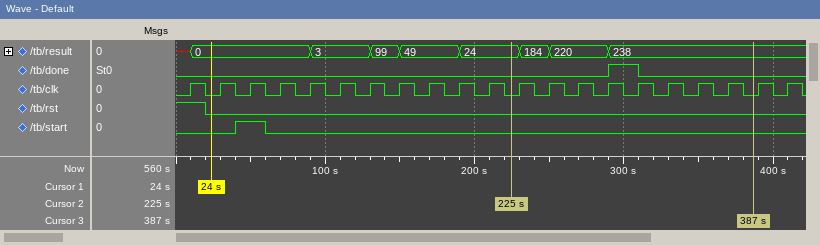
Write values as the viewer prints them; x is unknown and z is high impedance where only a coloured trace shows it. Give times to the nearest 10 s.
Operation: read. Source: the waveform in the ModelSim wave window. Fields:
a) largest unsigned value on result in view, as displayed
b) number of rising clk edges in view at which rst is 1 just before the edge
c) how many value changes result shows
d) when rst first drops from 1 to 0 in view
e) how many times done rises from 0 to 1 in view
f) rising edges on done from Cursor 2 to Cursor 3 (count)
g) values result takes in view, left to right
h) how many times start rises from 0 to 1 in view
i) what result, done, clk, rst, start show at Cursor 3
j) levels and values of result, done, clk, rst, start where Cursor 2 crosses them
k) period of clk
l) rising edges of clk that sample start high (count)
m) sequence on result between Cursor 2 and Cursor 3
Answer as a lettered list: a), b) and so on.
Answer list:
a) 238
b) 1
c) 8
d) 20 s
e) 1
f) 1
g) x, 0, 3, 99, 49, 24, 184, 220, 238
h) 1
i) result=238, done=0, clk=0, rst=0, start=0
j) result=24, done=0, clk=0, rst=0, start=0
k) 20 s
l) 1
m) 24, 184, 220, 238
